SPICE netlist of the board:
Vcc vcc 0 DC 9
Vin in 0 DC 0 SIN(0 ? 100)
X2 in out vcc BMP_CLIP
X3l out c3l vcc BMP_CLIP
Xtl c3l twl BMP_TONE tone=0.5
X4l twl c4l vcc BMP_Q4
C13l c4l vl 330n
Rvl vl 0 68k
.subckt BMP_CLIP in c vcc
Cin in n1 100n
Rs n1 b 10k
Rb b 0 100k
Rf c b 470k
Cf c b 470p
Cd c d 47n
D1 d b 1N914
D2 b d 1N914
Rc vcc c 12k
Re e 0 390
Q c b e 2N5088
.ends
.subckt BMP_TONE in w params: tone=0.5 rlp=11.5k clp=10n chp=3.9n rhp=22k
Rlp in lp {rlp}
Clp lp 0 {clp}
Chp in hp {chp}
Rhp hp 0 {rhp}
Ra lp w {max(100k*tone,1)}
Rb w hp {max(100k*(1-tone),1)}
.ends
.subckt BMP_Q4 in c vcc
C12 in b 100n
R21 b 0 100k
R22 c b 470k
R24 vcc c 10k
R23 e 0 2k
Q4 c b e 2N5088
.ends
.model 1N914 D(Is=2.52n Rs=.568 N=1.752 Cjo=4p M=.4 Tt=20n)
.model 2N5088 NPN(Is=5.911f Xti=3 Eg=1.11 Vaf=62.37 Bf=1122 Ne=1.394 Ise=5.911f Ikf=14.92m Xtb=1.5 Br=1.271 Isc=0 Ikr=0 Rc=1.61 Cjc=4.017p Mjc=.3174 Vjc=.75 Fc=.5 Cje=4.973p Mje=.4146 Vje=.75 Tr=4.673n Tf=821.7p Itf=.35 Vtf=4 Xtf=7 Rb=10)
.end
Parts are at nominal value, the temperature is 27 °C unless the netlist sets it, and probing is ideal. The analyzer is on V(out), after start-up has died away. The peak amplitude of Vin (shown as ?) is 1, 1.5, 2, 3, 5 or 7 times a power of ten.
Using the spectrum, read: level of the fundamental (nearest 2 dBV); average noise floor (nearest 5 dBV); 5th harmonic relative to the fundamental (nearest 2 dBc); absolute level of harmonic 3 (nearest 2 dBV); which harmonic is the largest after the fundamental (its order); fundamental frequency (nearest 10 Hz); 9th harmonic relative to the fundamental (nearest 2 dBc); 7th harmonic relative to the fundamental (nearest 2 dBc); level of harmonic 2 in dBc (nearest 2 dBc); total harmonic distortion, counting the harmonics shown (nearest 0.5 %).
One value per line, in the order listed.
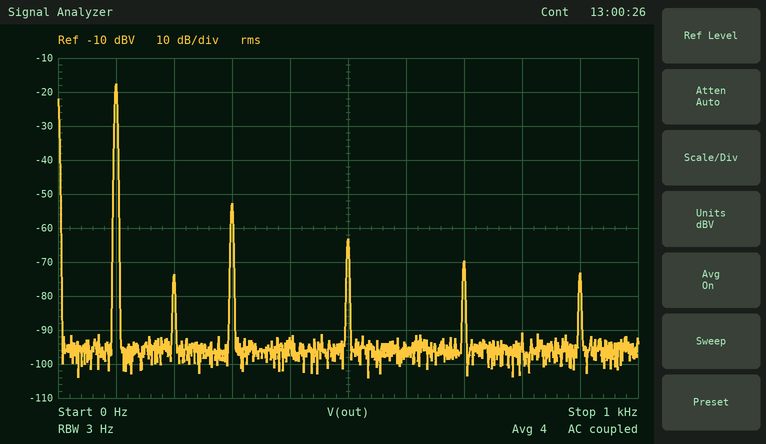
-18 dBV
-95 dBV
-46 dBc
-52 dBV
3
100 Hz
-56 dBc
-52 dBc
-56 dBc
2.0 %
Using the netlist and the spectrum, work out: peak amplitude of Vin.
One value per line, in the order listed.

20 mV
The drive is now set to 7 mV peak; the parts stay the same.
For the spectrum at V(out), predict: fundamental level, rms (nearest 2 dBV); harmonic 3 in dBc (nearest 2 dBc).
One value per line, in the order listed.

-26 dBV
-36 dBc
